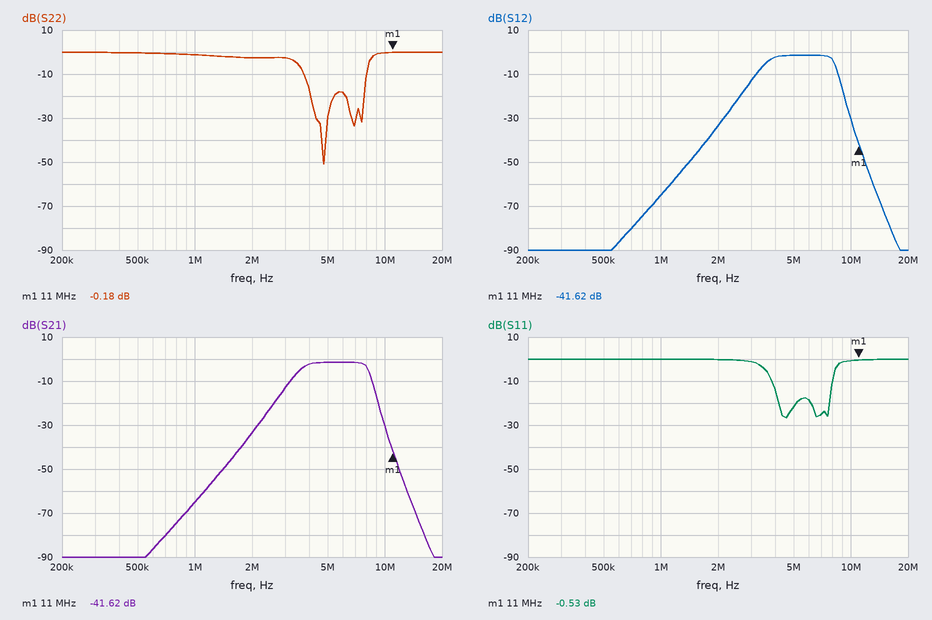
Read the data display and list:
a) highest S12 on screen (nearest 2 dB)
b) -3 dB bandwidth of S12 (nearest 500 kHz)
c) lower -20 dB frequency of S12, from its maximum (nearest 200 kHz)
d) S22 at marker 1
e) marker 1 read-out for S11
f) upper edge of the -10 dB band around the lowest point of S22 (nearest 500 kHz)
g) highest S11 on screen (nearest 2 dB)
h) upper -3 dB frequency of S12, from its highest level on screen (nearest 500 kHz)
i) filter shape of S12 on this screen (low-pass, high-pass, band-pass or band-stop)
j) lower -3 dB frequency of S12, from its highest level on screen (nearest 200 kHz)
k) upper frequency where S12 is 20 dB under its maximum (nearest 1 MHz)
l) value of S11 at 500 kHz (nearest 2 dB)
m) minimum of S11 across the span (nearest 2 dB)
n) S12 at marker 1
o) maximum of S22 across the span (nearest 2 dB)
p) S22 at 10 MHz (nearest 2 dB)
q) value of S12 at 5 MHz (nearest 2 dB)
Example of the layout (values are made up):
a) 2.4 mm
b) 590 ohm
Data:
a) -2 dB
b) 4.5 MHz
c) 2.6 MHz
d) -0.18 dB
e) -0.53 dB
f) 8.0 MHz
g) 0 dB
h) 8.0 MHz
i) band-pass
j) 3.6 MHz
k) 9 MHz
l) 0 dB
m) -26 dB
n) -41.62 dB
o) 0 dB
p) 0 dB
q) -2 dB
